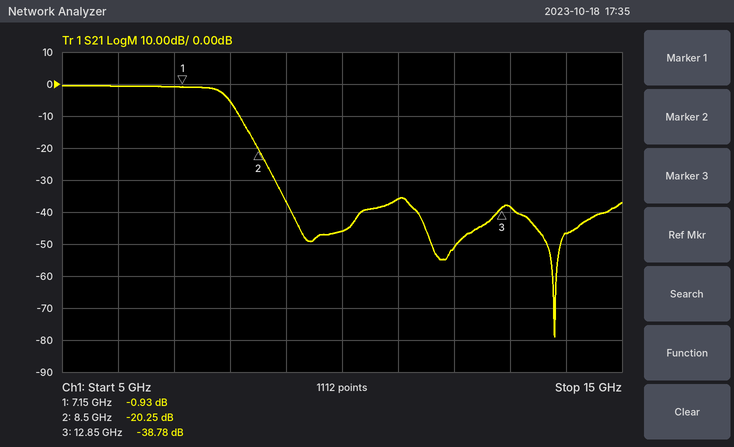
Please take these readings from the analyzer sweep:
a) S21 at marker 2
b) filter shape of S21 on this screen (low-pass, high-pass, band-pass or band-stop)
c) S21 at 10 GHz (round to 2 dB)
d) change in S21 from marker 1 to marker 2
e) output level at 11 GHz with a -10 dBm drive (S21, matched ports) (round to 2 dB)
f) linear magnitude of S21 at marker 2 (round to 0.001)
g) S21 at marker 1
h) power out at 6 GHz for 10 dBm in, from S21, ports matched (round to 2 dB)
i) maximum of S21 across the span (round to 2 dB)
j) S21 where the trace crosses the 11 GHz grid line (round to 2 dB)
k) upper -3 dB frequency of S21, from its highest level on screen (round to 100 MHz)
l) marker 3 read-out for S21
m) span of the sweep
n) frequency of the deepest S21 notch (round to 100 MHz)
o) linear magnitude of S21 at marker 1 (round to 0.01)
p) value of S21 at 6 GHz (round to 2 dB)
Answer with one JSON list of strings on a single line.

["-20.25 dB", "low-pass", "-46 dB", "-19.32 dB", "-46 dBm", "0.097", "-0.93 dB", "10 dBm", "0 dB", "-36 dB", "7.9 GHz", "-38.78 dB", "10 GHz", "13.8 GHz", "0.90", "0 dB"]
